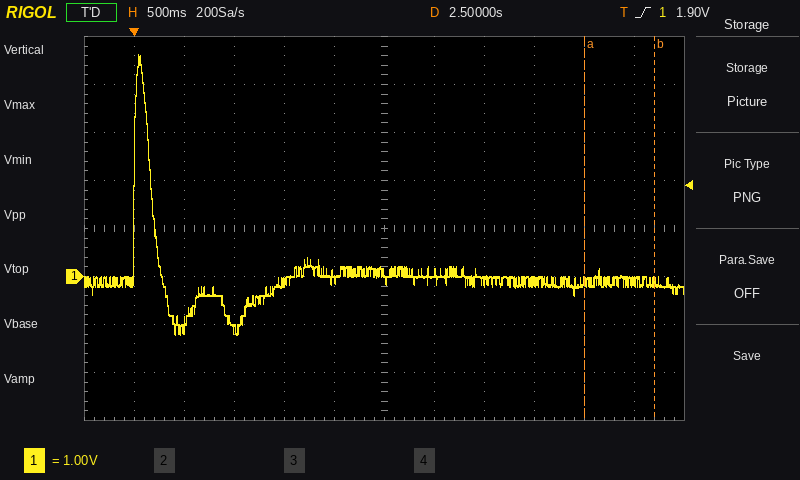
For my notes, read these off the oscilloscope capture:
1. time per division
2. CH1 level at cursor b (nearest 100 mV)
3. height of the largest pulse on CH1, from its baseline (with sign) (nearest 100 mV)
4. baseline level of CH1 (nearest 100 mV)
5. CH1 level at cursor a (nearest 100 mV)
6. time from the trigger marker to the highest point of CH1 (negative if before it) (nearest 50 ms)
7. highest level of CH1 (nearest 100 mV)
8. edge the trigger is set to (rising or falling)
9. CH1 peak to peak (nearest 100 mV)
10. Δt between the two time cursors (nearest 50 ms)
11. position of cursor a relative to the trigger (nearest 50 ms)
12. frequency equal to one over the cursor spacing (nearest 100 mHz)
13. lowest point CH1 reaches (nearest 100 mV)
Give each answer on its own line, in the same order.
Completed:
500 ms
-100 mV
+4.7 V
-100 mV
-100 mV
+50 ms
4.6 V
rising
5.8 V
700 ms
+4.50 s
1.4 Hz
-1.2 V
